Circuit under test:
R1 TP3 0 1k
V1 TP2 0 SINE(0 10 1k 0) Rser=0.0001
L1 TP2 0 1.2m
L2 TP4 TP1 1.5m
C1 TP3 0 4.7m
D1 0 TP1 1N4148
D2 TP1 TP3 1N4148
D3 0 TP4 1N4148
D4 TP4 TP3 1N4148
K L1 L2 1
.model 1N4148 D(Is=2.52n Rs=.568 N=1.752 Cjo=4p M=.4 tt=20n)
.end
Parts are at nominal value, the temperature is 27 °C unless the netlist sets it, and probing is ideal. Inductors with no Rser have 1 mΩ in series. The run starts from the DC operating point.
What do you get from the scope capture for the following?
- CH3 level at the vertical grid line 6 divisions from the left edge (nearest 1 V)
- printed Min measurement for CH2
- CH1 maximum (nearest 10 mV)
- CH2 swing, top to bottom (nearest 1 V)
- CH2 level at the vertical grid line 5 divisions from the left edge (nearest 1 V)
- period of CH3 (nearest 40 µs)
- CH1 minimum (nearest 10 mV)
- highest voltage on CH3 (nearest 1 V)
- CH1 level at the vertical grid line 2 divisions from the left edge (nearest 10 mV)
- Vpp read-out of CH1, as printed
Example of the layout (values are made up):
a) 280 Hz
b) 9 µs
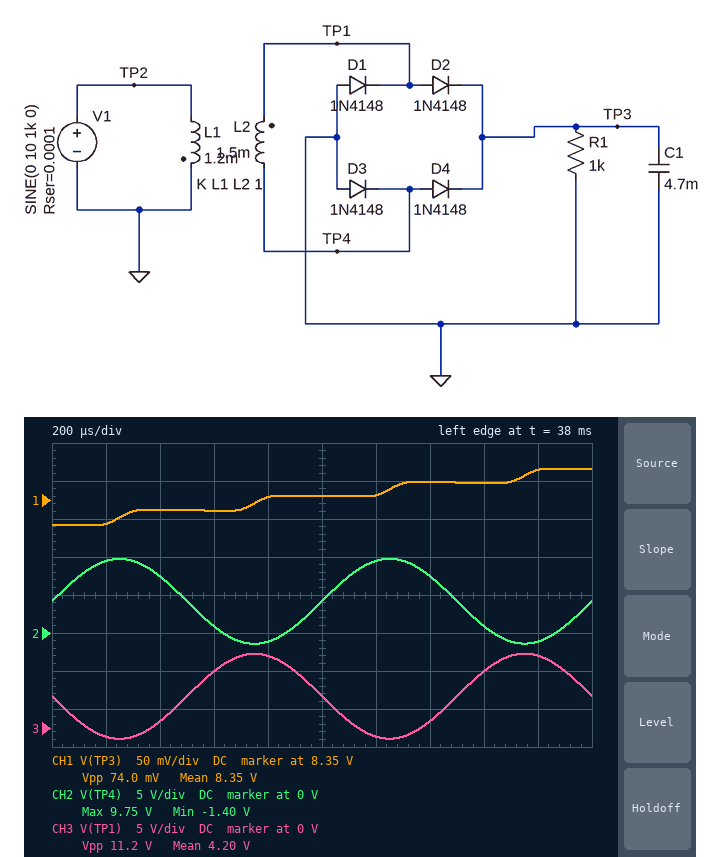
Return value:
a) -1 V
b) -1.40 V
c) 8.39 V
d) 11 V
e) 4 V
f) 1.00 ms
g) 8.32 V
h) 10 V
i) 8.34 V
j) 74.0 mV
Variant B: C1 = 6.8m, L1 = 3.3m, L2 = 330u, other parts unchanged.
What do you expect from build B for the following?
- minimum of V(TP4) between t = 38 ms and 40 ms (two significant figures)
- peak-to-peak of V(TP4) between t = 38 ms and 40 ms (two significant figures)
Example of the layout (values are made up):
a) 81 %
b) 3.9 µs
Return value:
a) -1.0 V
b) 3.2 V
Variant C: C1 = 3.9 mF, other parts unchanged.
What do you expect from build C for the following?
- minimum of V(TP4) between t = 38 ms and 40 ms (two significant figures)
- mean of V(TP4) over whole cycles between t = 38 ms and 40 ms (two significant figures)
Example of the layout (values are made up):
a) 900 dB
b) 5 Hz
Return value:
a) -1.3 V
b) 4.3 V
